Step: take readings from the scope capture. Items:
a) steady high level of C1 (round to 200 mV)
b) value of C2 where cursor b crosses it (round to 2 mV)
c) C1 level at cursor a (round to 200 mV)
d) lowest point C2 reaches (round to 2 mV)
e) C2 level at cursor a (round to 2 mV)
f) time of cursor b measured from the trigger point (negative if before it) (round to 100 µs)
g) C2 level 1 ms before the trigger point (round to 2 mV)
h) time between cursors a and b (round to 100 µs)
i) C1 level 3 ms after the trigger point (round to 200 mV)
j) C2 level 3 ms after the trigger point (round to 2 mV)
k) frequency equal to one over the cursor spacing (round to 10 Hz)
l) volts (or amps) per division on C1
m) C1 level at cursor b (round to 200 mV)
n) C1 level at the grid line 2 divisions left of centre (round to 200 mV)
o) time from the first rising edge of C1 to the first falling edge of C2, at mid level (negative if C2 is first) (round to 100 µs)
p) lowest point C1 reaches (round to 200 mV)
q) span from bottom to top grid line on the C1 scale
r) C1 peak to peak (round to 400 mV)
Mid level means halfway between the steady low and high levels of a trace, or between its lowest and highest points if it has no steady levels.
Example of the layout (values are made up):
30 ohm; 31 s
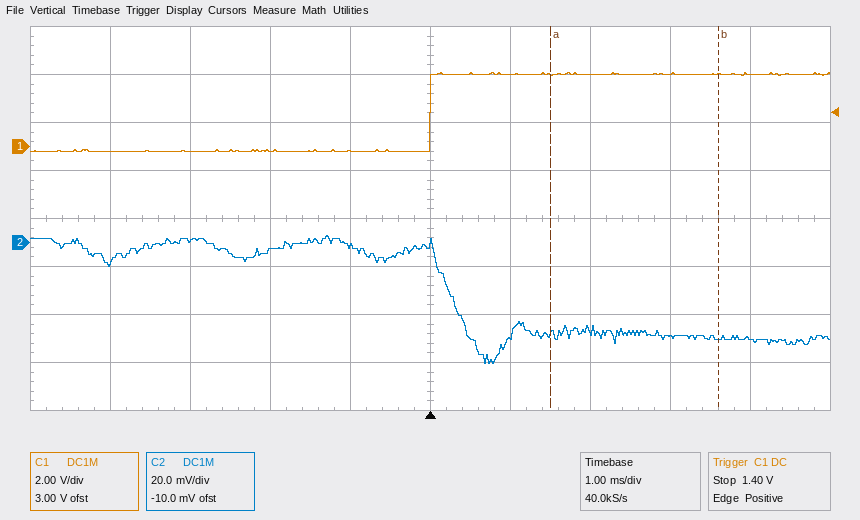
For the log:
3.0 V; -40 mV; 3.0 V; -50 mV; -38 mV; +3.6 ms; -2 mV; 2.1 ms; 3.0 V; -40 mV; 480 Hz; 2 V; 3.0 V; -200 mV; +300 µs; -200 mV; 16 V; 3.2 V
